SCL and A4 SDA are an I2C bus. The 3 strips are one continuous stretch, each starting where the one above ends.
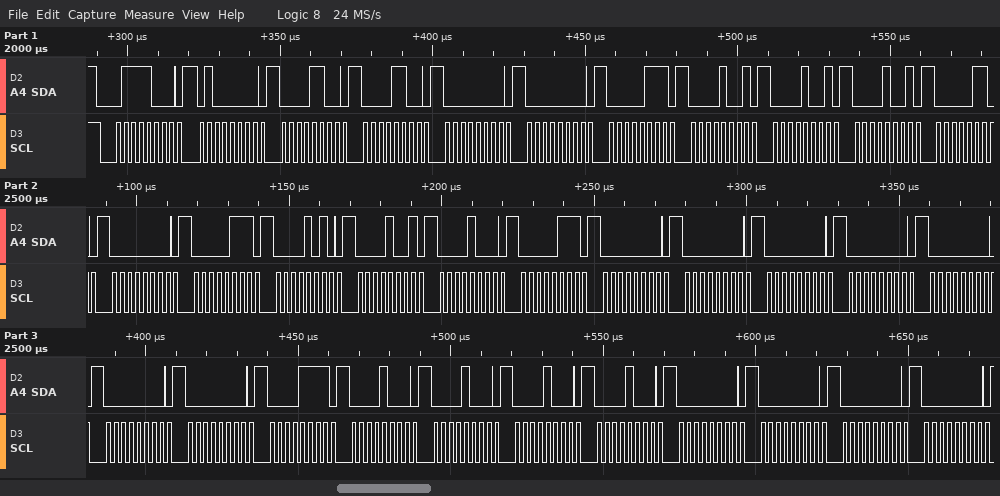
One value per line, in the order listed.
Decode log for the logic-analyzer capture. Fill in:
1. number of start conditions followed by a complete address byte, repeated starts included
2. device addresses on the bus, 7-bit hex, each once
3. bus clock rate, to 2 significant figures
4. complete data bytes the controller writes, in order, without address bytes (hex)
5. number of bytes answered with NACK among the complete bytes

1
0x3C
400 kHz
40 0C 0C 00 00 07 09 09 09 06 00 07 0A 09 08 07 00 00 00 00 00 00 00 0F 08 08 08 08 00 00 00 00
0
